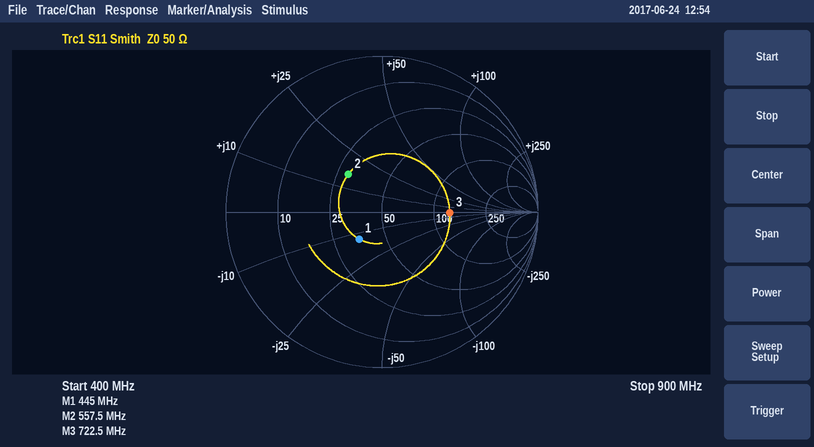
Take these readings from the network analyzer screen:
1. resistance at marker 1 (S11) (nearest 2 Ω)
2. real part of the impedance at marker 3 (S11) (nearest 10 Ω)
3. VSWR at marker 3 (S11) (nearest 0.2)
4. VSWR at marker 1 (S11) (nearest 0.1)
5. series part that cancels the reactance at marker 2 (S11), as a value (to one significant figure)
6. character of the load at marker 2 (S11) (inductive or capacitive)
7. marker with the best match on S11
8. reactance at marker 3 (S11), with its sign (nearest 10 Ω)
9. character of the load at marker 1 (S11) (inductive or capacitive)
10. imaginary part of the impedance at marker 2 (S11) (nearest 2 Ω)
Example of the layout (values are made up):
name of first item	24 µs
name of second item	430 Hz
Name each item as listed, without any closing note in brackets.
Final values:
resistance at marker 1 (S11)	36 Ω
real part of the impedance at marker 3 (S11)	130 Ω
VSWR at marker 3 (S11)	2.6
VSWR at marker 1 (S11)	1.6
series part that cancels the reactance at marker 2 (S11), as a value	20 pF
character of the load at marker 2 (S11)	inductive
marker with the best match on S11	marker 1
reactance at marker 3 (S11), with its sign	0 Ω
character of the load at marker 1 (S11)	capacitive
imaginary part of the impedance at marker 2 (S11)	+16 Ω
